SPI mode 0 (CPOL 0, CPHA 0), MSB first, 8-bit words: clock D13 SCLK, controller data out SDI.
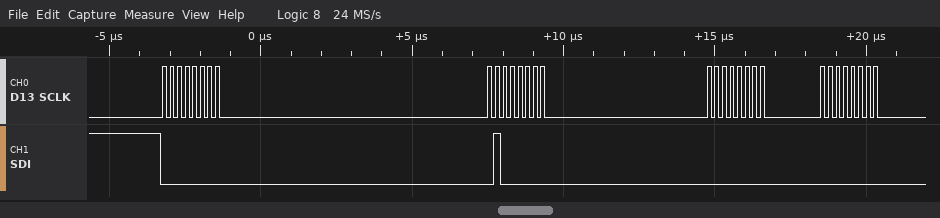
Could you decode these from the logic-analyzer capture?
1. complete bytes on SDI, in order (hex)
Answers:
00 40 00 00
